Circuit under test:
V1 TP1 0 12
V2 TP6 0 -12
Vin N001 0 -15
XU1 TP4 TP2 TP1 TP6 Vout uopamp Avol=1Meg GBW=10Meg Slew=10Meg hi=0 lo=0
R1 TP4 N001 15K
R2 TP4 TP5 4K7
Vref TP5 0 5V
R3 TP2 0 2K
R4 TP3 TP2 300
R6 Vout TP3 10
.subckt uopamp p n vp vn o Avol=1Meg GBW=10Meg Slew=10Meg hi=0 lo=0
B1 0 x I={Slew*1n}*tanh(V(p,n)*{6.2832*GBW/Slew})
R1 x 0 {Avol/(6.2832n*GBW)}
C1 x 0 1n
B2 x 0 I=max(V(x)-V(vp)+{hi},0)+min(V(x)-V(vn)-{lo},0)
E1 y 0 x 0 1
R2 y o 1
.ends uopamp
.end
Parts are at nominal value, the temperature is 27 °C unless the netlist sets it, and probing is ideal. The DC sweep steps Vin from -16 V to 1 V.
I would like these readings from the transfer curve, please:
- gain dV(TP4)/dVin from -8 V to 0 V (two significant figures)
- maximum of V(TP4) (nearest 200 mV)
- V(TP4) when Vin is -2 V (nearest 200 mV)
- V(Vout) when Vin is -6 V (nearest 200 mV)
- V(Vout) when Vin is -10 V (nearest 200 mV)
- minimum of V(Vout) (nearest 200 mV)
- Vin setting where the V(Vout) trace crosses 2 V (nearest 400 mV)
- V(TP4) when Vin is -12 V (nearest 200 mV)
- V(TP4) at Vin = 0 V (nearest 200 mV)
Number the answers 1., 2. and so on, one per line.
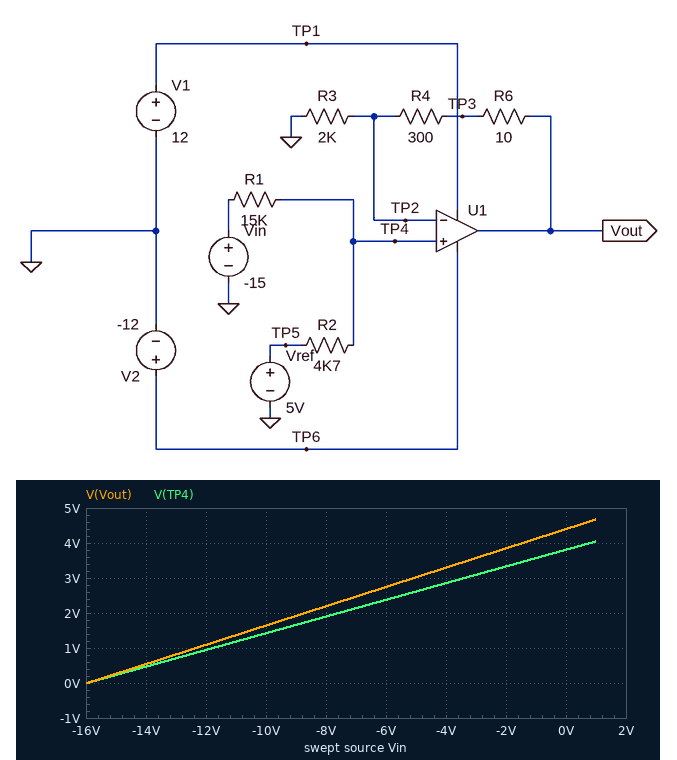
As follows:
1. 0.24 V/V
2. 4.0 V
3. 3.4 V
4. 2.8 V
5. 1.6 V
6. 0 V
7. -8.8 V
8. 1.0 V
9. 3.8 V
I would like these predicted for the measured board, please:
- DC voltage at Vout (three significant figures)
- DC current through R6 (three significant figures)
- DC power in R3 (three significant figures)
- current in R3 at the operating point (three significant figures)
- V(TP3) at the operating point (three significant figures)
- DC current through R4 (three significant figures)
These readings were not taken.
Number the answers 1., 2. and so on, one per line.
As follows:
1. 264 mV
2. 114 µA
3. 26.1 µW
4. 114 µA
5. 263 mV
6. 114 µA
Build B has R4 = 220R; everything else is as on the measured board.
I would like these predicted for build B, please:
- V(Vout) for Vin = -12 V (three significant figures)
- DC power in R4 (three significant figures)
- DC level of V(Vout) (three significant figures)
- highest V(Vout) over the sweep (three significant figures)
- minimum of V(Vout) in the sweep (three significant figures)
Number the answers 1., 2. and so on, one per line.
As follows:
1. 1.05 V
2. 2.87 µW
3. 255 mV
4. 4.51 V
5. -11.3 mV
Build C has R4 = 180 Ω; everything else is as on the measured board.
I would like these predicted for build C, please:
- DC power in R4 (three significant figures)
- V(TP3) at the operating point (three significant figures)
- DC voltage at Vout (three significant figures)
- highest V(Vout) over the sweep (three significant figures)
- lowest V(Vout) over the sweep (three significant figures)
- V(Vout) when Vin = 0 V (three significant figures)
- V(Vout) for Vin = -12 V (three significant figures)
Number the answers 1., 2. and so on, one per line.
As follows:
1. 2.35 µW
2. 249 mV
3. 250 mV
4. 4.43 V
5. -11.1 mV
6. 4.17 V
7. 1.03 V
